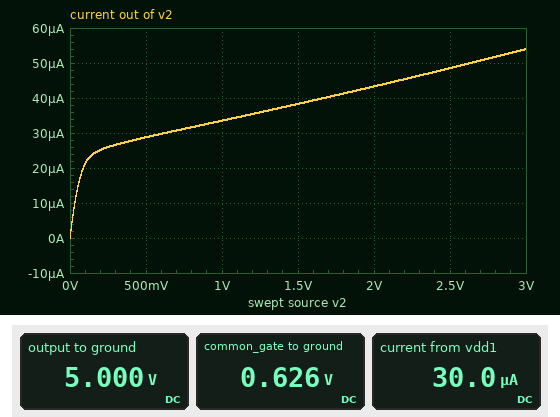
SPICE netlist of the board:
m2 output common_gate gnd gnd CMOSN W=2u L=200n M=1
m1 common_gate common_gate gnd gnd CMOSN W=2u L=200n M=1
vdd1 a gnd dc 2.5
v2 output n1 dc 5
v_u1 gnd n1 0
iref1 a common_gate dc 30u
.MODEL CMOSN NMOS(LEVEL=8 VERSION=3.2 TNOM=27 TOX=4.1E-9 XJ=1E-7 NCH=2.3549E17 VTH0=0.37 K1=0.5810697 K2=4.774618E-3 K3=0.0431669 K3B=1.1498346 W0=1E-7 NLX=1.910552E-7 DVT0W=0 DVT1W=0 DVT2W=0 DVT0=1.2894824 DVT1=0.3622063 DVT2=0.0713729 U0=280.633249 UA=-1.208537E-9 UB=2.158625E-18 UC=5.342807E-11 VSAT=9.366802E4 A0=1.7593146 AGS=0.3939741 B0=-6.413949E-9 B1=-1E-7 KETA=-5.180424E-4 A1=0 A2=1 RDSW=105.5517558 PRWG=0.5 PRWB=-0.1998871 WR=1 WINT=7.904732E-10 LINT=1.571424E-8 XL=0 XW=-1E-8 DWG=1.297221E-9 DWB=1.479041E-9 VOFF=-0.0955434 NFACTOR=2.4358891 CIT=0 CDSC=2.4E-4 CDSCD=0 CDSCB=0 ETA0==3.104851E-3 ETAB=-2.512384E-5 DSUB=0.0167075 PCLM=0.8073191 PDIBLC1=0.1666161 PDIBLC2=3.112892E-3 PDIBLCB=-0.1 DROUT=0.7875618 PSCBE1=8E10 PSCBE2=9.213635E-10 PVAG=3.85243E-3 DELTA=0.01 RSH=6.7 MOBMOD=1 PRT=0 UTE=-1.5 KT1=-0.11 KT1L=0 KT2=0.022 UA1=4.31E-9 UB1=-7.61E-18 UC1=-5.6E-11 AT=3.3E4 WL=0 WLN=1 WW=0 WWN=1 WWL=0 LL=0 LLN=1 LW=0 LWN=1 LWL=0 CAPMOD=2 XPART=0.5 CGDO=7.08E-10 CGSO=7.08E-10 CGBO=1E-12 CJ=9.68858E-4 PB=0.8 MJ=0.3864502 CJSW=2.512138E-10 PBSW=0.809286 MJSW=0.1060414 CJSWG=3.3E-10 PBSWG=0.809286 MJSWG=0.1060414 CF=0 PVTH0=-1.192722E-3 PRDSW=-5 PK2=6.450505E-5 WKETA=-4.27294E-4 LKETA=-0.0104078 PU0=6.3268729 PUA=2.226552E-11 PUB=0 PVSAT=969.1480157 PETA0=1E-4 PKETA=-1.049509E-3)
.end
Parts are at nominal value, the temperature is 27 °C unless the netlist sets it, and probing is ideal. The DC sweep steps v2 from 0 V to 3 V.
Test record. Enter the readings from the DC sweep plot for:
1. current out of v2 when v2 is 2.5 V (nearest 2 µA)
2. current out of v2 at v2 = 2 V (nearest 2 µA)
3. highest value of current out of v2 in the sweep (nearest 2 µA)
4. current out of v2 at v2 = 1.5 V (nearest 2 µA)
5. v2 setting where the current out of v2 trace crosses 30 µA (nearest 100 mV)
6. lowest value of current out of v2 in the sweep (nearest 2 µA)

48 µA
44 µA
54 µA
38 µA
600 mV
0 A
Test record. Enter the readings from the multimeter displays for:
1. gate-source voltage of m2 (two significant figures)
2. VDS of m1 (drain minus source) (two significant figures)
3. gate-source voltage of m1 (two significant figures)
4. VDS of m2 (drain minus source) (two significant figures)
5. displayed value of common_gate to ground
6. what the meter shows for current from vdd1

630 mV
630 mV
630 mV
5.0 V
0.626 V
30.0 µA
